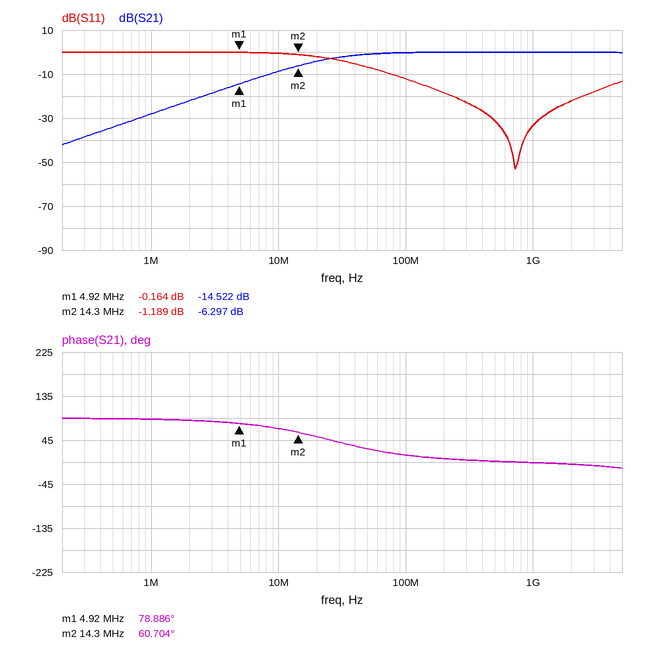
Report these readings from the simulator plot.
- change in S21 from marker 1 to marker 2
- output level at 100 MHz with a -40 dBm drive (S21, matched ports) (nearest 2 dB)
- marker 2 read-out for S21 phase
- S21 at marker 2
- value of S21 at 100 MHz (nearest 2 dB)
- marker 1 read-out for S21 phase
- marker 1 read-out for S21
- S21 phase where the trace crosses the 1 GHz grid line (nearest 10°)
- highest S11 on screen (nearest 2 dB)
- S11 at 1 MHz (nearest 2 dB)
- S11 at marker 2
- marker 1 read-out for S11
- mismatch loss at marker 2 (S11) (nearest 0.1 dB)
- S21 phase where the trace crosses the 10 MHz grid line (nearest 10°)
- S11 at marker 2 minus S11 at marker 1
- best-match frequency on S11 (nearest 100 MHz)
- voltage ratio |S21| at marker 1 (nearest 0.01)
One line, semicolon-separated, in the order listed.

8.225 dB; -40 dBm; 60.704°; -6.297 dB; 0 dB; 78.886°; -14.522 dB; 0°; 0 dB; 0 dB; -1.189 dB; -0.164 dB; 6.2 dB; 70°; -1.025 dB; 700 MHz; 0.19
